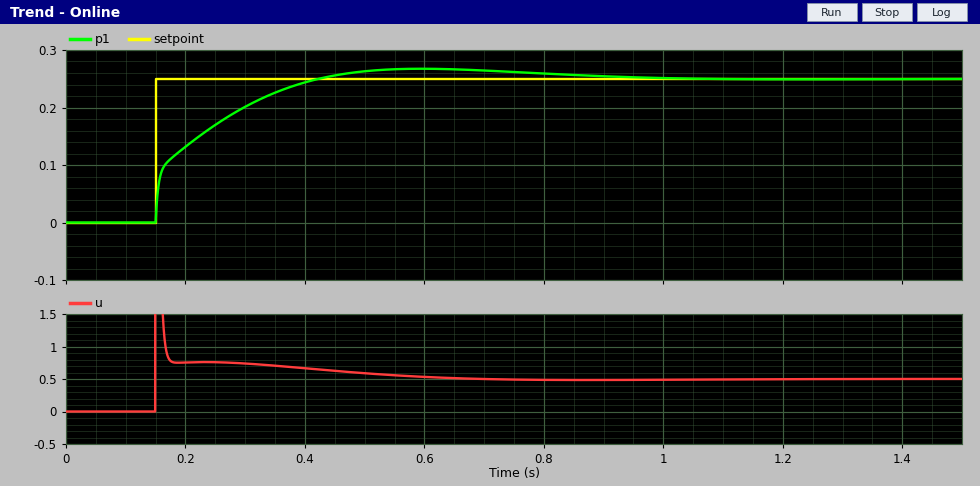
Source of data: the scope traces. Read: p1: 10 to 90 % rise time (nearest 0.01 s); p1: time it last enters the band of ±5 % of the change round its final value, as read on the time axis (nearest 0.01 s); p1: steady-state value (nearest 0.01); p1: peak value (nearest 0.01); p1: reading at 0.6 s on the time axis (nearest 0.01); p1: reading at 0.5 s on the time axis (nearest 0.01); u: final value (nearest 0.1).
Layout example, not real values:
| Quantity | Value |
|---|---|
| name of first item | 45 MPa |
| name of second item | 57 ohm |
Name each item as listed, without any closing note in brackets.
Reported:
| Quantity | Value |
|---|---|
| p1: 10 to 90 % rise time | 0.20 s |
| p1: time it last enters the band of ±5 % of the change round its final value, as read on the time axis | 0.74 s |
| p1: steady-state value | 0.25 |
| p1: peak value | 0.27 |
| p1: reading at 0.6 s on the time axis | 0.27 |
| p1: reading at 0.5 s on the time axis | 0.26 |
| u: final value | 0.5 |
